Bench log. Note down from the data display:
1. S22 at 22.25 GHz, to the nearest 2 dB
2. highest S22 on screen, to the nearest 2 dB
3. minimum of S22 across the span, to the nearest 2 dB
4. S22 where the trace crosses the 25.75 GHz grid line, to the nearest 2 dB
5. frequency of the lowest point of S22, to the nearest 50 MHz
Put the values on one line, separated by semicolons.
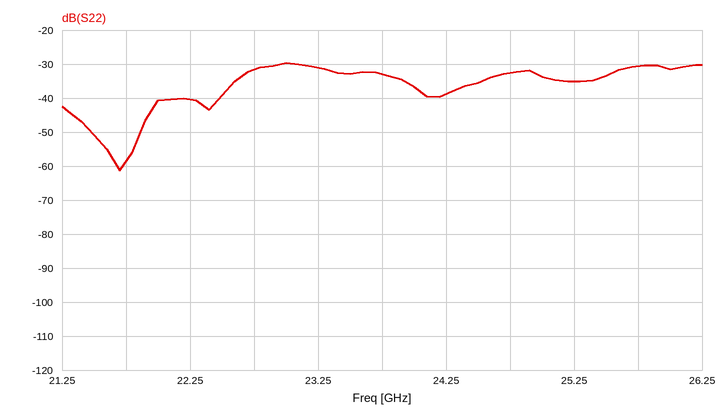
-40 dB; -30 dB; -62 dB; -30 dB; 21.70 GHz
